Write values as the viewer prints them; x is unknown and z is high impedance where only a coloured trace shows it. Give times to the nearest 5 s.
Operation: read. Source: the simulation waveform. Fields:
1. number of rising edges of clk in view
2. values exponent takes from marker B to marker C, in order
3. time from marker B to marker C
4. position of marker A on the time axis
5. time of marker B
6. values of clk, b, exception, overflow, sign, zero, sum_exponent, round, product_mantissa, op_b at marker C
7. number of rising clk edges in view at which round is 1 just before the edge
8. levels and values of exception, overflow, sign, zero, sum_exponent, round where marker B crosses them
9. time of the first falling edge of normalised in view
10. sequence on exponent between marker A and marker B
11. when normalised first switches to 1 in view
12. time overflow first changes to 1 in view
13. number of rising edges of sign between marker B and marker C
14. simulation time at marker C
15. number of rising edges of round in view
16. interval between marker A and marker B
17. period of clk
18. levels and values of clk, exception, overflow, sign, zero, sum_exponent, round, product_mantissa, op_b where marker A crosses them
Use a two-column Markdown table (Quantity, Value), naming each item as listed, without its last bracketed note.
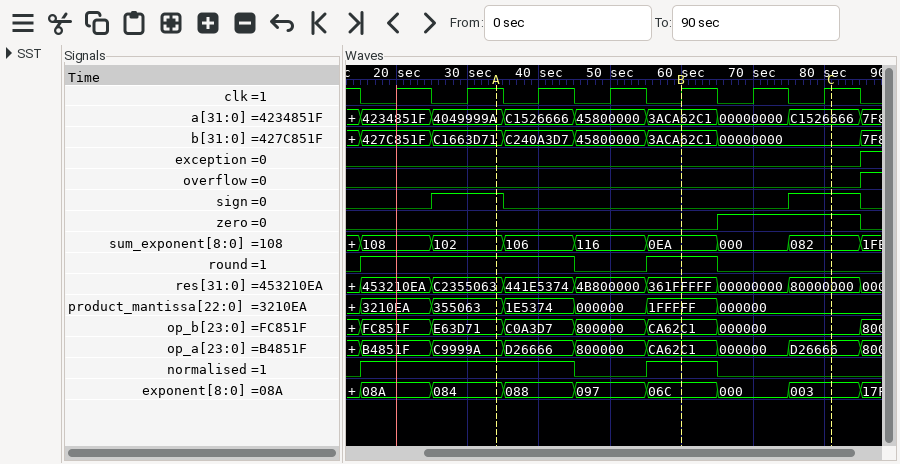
| Quantity | Value |
|---|---|
| number of rising edges of clk in view | 7 |
| values exponent takes from marker B to marker C, in order | 06C, 000, 003 |
| time from marker B to marker C | 20 s |
| position of marker A on the time axis | 35 s |
| time of marker B | 60 s |
| values of clk, b, exception, overflow, sign, zero, sum_exponent, round, product_mantissa, op_b at marker C | clk=1, b=00000000, exception=0, overflow=0, sign=1, zero=1, sum_exponent=082, round=0, product_mantissa=000000, op_b=000000 |
| number of rising clk edges in view at which round is 1 just before the edge | 4 |
| levels and values of exception, overflow, sign, zero, sum_exponent, round where marker B crosses them | exception=0, overflow=0, sign=0, zero=0, sum_exponent=0EA, round=1 |
| time of the first falling edge of normalised in view | 45 s |
| sequence on exponent between marker A and marker B | 084, 088, 097, 06C |
| when normalised first switches to 1 in view | 15 s |
| time overflow first changes to 1 in view | 85 s |
| number of rising edges of sign between marker B and marker C | 1 |
| simulation time at marker C | 80 s |
| number of rising edges of round in view | 2 |
| interval between marker A and marker B | 25 s |
| period of clk | 10 s |
| levels and values of clk, exception, overflow, sign, zero, sum_exponent, round, product_mantissa, op_b where marker A crosses them | clk=1, exception=0, overflow=0, sign=1, zero=0, sum_exponent=102, round=1, product_mantissa=355063, op_b=E63D71 |
